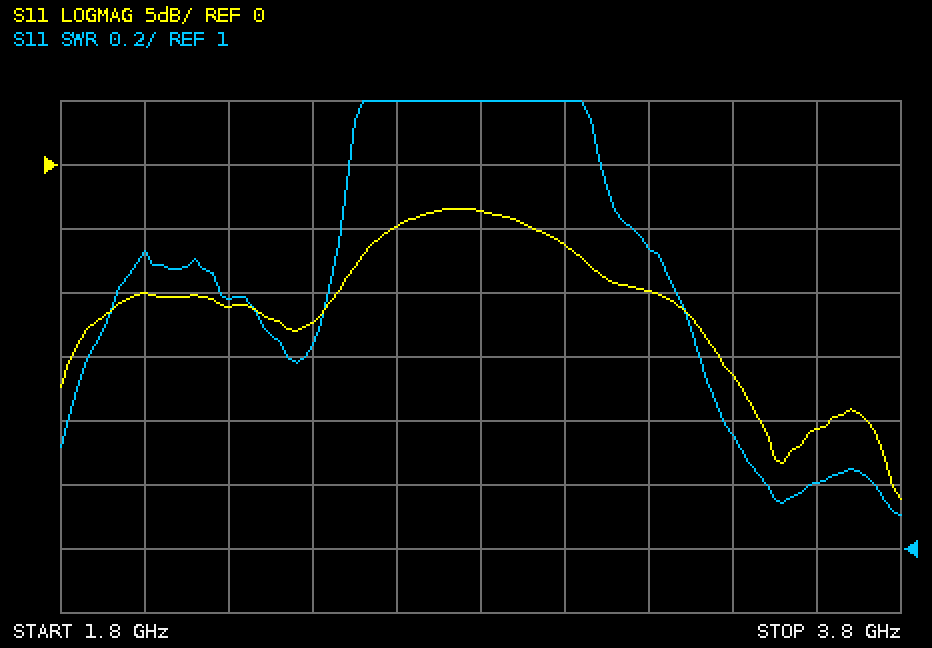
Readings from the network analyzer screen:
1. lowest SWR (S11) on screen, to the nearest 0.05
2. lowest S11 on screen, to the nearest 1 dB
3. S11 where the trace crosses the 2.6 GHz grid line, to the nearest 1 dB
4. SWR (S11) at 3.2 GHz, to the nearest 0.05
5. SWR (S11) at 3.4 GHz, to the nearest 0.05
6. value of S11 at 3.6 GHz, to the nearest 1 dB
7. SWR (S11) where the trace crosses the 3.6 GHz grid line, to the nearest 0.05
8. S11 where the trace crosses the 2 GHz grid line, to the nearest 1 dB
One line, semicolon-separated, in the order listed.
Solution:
1.10; -26 dB; -5 dB; 1.95; 1.35; -21 dB; 1.20; -10 dB
